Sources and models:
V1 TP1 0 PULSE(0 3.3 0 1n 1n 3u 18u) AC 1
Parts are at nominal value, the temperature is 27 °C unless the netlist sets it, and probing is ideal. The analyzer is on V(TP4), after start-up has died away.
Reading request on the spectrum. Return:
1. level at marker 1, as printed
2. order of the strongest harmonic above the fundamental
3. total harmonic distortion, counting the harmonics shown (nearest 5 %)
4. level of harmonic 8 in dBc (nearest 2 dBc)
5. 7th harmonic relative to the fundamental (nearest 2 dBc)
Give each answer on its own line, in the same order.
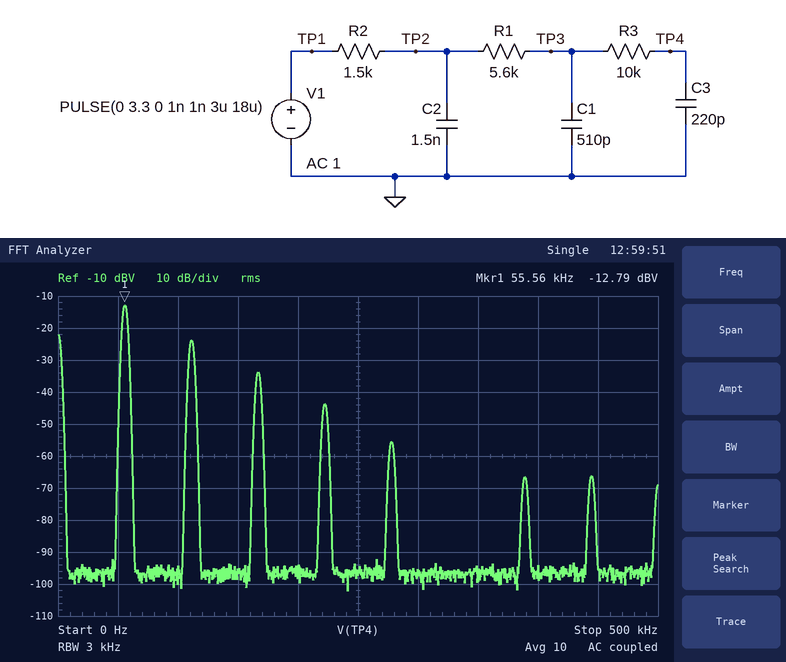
-12.79 dBV
2
30 %
-54 dBc
-54 dBc
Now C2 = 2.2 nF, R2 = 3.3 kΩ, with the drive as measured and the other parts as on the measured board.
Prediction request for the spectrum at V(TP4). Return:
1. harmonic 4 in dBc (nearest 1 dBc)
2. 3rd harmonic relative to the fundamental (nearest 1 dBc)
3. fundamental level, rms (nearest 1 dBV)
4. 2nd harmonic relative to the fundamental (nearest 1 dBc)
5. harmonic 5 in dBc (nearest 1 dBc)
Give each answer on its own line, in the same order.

-34 dBc
-24 dBc
-19 dBV
-13 dBc
-46 dBc
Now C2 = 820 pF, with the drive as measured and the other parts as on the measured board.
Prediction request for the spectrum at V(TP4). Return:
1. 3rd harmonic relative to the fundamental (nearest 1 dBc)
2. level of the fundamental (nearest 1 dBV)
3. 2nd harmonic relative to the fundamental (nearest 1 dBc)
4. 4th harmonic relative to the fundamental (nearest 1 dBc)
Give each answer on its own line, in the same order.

-19 dBc
-12 dBV
-10 dBc
-28 dBc
